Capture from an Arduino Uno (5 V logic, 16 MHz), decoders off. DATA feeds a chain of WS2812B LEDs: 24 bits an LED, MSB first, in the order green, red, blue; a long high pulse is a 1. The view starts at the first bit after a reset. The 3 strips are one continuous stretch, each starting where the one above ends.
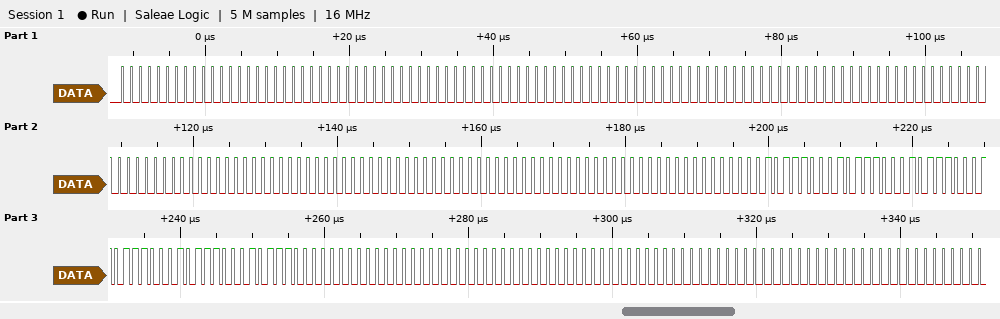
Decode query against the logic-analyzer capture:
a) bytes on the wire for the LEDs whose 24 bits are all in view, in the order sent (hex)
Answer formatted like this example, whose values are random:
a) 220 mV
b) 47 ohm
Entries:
a) 00 00 00 00 00 00 00 00 00 00 00 00 00 00 00 00 00 00 00 00 00 5C 5C 5C 5C 5C 5C 00 00 00 00 00 00 00 00 00
